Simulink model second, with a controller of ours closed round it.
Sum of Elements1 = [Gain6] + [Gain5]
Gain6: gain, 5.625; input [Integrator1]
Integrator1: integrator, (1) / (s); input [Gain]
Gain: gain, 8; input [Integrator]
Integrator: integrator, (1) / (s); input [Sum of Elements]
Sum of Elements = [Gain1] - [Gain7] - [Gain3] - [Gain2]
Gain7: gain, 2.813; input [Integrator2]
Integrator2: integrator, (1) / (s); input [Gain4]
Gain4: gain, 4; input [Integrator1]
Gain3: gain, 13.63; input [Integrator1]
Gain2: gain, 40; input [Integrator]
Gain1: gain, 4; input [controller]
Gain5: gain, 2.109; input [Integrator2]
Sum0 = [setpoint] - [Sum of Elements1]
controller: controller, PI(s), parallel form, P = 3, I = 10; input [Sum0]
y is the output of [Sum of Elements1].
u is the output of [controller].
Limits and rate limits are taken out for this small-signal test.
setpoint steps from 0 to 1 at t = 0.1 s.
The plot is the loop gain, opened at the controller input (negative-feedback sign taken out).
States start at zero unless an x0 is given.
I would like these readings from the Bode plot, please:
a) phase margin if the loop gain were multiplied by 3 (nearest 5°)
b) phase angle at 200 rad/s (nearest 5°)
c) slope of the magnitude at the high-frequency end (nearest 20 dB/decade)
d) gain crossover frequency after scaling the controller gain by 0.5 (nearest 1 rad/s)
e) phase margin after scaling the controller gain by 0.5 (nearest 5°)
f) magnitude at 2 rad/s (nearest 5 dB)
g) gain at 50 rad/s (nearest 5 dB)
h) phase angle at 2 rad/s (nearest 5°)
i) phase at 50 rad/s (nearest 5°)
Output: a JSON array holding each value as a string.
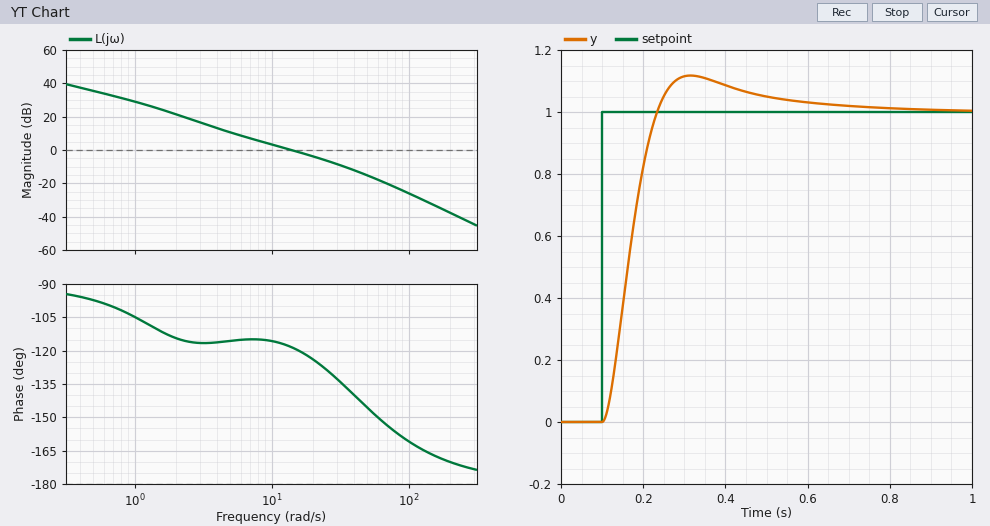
["45°", "-170°", "-40 dB/decade", "8 rad/s", "65°", "20 dB", "-15 dB", "-115°", "-145°"]
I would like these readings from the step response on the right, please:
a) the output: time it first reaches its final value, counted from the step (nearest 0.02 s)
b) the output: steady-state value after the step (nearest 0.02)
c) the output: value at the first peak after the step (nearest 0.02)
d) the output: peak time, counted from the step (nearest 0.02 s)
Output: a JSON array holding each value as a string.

["0.14 s", "1.00", "1.12", "0.22 s"]
